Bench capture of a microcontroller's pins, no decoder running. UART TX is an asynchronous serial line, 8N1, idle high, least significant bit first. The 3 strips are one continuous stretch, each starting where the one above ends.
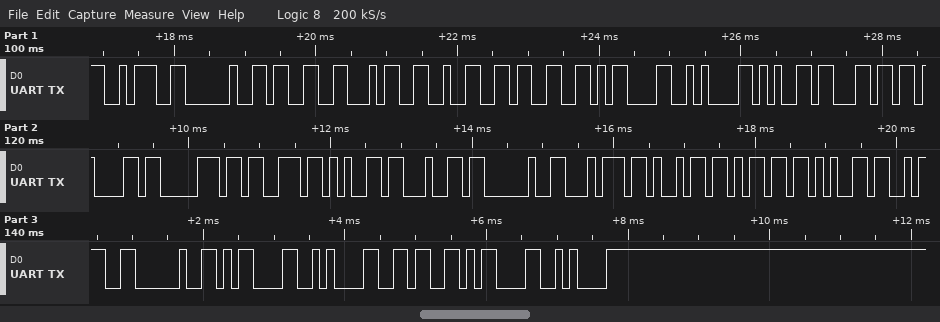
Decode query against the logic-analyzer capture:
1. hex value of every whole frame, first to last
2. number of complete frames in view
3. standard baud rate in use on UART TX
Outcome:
3A 20 33 34 32 33 0D 0A 65 6C 61 70 73 65 64 20 74 69 6D 65 3A 20 0D 0A 36 0D 0A
27
9600 baud
